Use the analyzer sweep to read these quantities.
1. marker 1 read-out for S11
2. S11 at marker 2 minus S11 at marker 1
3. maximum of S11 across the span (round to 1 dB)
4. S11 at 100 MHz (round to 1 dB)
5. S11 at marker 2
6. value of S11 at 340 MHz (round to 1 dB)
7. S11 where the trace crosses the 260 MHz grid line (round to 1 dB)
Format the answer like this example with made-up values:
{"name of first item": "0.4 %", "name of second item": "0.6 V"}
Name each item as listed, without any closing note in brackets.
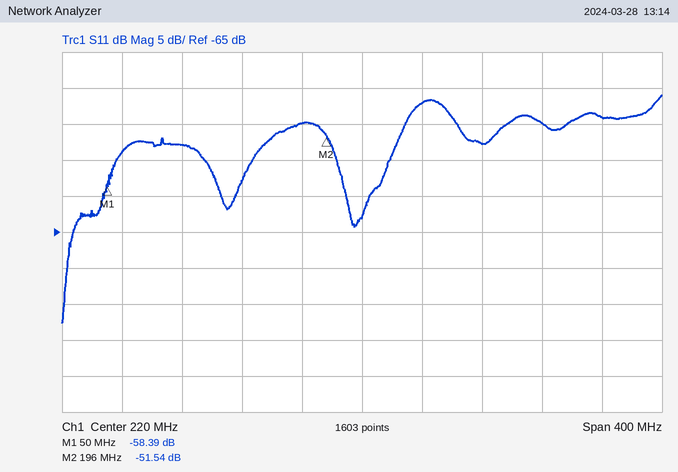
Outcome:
{"marker 1 read-out for S11": "-58.39 dB", "S11 at marker 2 minus S11 at marker 1": "6.85 dB", "maximum of S11 across the span": "-46 dB", "S11 at 100 MHz": "-53 dB", "S11 at marker 2": "-51.54 dB", "value of S11 at 340 MHz": "-50 dB", "S11 where the trace crosses the 260 MHz grid line": "-47 dB"}
